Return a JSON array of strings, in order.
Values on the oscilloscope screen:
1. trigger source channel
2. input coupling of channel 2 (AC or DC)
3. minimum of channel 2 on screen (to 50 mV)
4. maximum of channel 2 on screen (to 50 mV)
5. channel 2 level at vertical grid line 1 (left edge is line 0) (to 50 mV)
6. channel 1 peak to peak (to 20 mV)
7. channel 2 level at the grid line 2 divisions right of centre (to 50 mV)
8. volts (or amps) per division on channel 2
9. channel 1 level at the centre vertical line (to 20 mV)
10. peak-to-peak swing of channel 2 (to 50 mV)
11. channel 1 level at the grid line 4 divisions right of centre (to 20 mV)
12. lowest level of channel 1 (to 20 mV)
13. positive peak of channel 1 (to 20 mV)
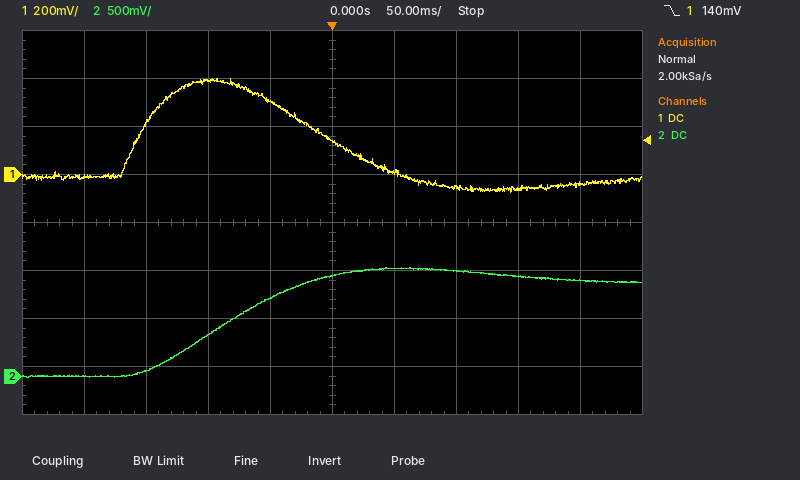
["channel 1", "DC", "0 mV", "1.15 V", "0 mV", "480 mV", "1.10 V", "500 mV", "140 mV", "1.15 V", "-40 mV", "-80 mV", "400 mV"]
